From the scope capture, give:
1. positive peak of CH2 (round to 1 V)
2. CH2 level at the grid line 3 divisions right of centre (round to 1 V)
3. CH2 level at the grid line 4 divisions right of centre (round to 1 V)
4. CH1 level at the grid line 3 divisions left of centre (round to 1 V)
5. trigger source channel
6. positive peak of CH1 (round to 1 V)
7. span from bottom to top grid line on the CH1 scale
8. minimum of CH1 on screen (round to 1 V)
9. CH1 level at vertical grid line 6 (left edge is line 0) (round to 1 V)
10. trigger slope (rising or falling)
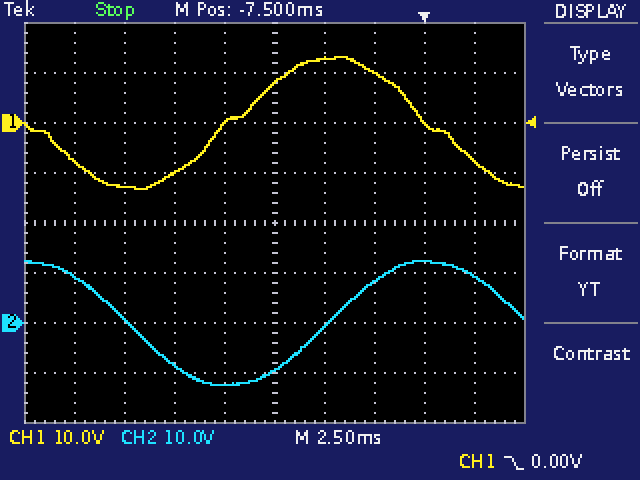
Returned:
12 V
12 V
9 V
-13 V
CH1
13 V
80 V
-13 V
13 V
falling
